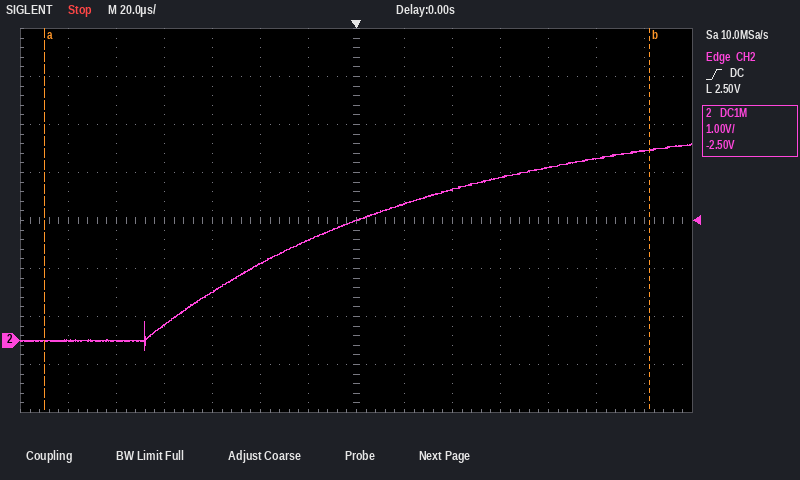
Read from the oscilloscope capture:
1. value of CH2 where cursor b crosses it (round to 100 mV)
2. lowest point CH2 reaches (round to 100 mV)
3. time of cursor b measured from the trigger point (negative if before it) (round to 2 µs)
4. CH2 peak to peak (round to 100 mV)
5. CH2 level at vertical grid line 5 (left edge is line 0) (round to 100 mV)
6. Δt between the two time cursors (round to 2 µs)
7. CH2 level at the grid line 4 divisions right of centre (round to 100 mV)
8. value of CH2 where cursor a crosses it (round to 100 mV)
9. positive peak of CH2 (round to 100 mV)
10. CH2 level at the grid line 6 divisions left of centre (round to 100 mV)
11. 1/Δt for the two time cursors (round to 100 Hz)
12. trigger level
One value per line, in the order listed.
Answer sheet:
4.0 V
-200 mV
+122 µs
4.3 V
1.6 V
252 µs
3.6 V
0.0 V
4.1 V
0.0 V
4.0 kHz
2.50 V
